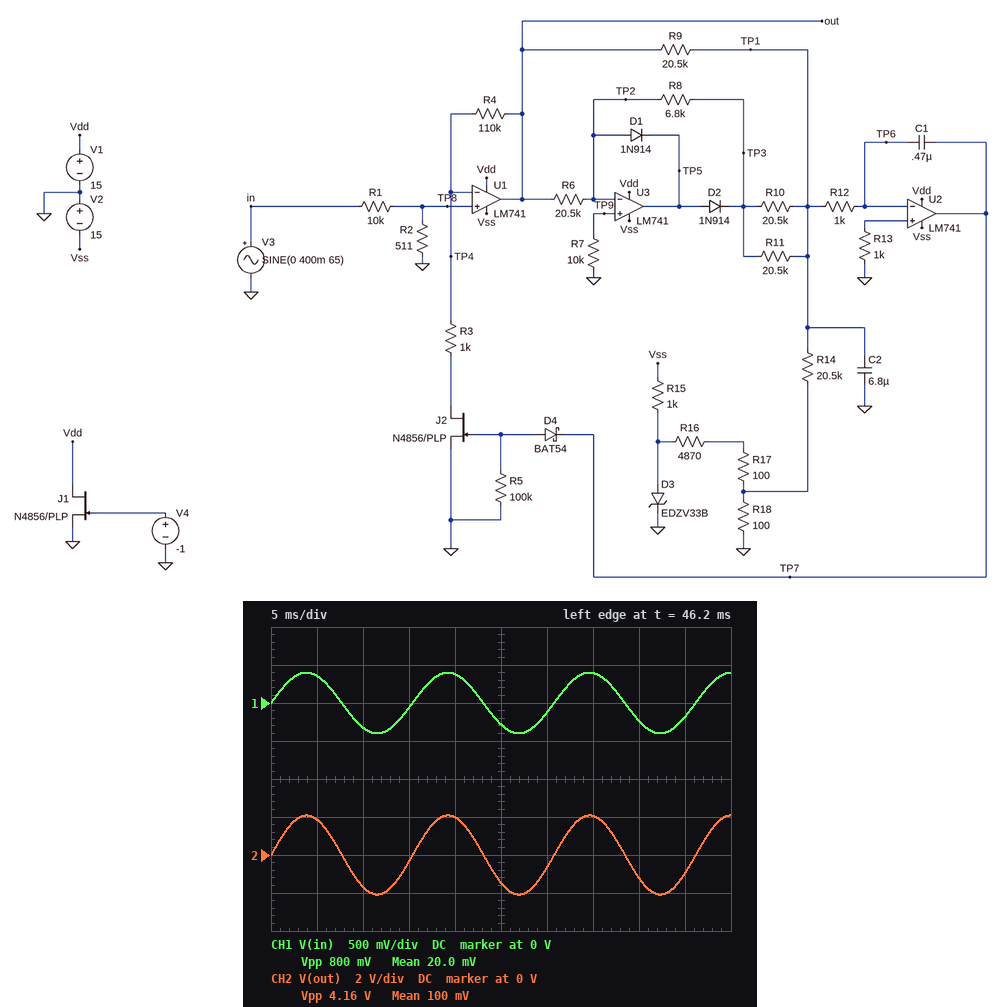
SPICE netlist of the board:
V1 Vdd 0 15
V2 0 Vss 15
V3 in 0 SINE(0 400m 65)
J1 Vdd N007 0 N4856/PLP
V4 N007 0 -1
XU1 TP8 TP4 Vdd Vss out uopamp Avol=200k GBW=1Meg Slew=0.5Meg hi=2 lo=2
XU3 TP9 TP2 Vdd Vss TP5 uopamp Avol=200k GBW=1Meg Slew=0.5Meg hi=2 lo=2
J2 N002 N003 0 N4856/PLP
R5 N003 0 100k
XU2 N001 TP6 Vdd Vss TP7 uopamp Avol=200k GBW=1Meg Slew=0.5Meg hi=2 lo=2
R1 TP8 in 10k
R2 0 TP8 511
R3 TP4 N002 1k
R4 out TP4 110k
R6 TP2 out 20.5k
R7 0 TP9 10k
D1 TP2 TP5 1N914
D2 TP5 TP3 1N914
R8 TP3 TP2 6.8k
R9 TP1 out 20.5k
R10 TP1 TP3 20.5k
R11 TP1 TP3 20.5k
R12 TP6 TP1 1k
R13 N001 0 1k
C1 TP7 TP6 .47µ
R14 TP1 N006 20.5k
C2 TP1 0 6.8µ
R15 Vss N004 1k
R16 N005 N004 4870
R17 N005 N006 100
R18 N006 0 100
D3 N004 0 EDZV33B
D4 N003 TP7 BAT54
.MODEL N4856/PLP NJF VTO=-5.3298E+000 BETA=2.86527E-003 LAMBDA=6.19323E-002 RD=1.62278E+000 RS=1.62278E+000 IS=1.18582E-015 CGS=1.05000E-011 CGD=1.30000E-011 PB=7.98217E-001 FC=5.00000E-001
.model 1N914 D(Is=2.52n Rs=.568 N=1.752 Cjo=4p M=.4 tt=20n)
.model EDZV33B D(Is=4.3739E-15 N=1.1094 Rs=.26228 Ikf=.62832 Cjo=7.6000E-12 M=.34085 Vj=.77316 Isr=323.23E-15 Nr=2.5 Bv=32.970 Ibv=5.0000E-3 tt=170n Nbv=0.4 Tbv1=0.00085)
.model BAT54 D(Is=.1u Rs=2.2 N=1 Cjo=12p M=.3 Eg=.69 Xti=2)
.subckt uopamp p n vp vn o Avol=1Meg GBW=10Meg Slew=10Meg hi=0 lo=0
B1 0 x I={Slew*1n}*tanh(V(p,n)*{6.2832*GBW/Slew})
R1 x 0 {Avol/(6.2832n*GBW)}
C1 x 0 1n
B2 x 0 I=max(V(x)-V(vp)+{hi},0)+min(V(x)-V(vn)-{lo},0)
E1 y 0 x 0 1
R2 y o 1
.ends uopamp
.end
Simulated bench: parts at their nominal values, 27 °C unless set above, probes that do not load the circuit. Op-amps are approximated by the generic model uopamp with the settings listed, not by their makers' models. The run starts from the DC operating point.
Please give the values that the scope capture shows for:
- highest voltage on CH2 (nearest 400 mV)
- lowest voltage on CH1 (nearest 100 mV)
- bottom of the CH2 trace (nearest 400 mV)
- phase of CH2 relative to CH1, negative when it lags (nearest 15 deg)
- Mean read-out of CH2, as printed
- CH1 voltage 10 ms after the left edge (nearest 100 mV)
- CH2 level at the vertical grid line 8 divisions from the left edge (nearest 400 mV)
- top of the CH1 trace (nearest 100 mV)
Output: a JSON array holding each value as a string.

["2.0 V", "-400 mV", "-2.0 V", "0 deg", "100 mV", "-300 mV", "-1.2 V", "400 mV"]
